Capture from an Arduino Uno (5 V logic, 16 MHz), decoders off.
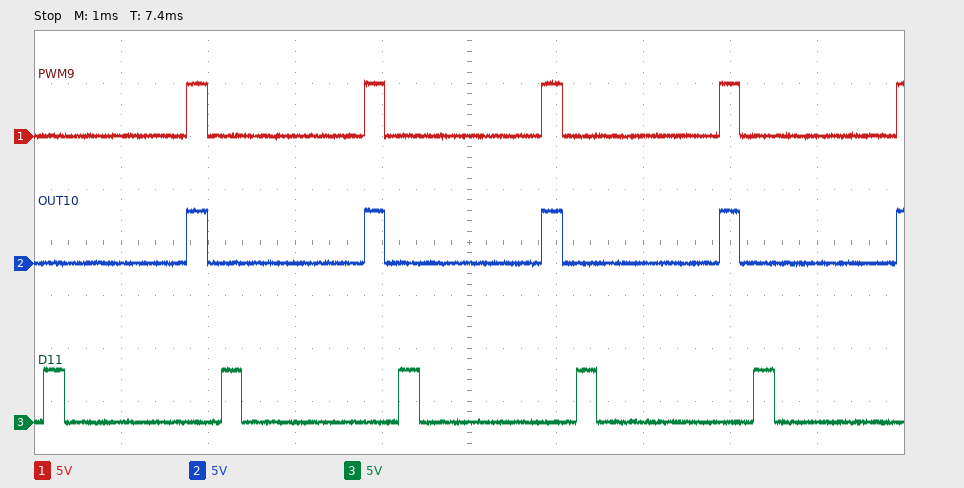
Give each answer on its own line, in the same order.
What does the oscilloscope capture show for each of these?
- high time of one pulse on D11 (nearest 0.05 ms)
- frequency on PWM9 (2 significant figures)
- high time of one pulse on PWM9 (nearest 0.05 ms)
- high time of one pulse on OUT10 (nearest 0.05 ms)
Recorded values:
0.25 ms
490 Hz
0.25 ms
0.25 ms
